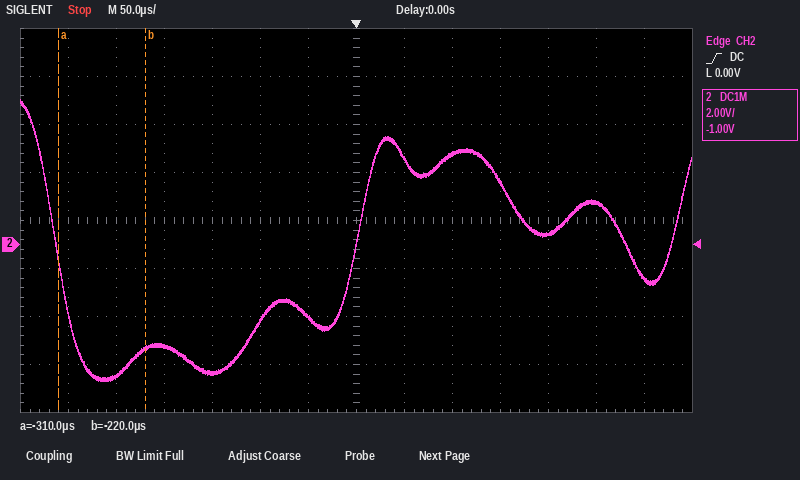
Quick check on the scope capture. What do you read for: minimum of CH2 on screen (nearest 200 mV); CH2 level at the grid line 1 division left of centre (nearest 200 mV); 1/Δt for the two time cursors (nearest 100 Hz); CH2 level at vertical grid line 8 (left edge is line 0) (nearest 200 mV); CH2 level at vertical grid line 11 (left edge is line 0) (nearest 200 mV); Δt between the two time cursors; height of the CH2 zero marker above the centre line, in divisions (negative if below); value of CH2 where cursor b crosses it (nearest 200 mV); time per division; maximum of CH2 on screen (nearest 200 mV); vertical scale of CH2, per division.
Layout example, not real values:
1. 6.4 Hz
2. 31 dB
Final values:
1. -5.6 V
2. -3.0 V
3. 11.1 kHz
4. 3.6 V
5. 400 mV
6. 90 µs
7. -0.5 div
8. -4.4 V
9. 50 µs
10. 6.0 V
11. 2 V
